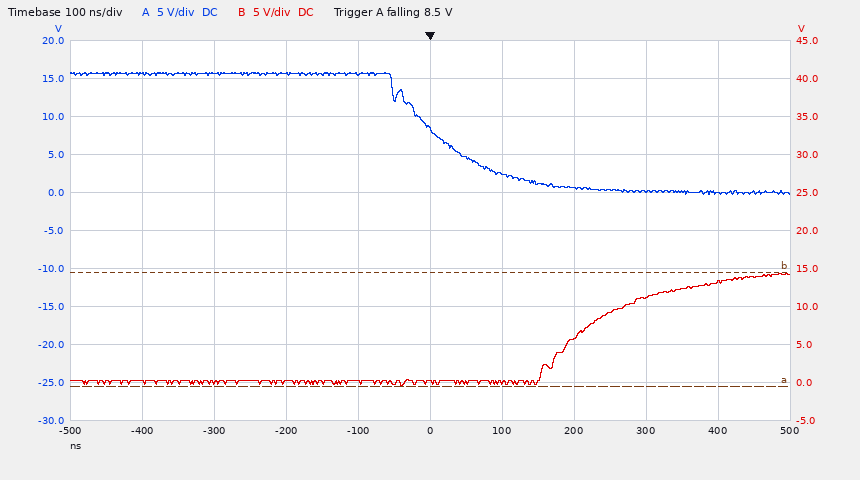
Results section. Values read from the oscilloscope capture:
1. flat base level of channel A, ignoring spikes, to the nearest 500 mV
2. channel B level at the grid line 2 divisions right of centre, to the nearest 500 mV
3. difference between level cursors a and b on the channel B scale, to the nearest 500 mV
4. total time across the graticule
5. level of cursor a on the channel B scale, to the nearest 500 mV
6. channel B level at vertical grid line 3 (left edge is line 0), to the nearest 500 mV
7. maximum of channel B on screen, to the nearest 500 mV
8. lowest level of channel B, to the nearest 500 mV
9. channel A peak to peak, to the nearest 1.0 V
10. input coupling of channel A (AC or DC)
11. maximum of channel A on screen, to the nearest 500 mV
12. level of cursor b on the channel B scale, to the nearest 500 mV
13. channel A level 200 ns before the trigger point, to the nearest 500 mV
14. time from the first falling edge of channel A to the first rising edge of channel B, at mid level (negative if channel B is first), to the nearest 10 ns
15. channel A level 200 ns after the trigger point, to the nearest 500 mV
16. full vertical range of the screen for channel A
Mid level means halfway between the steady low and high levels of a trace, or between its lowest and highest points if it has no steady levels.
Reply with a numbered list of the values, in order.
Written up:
1. 0.0 V
2. 6.0 V
3. 15.0 V
4. 1 µs
5. -500 mV
6. 0.0 V
7. 14.5 V
8. -500 mV
9. 16.0 V
10. DC
11. 16.0 V
12. 14.5 V
13. 15.5 V
14. +210 ns
15. 500 mV
16. 50 V
